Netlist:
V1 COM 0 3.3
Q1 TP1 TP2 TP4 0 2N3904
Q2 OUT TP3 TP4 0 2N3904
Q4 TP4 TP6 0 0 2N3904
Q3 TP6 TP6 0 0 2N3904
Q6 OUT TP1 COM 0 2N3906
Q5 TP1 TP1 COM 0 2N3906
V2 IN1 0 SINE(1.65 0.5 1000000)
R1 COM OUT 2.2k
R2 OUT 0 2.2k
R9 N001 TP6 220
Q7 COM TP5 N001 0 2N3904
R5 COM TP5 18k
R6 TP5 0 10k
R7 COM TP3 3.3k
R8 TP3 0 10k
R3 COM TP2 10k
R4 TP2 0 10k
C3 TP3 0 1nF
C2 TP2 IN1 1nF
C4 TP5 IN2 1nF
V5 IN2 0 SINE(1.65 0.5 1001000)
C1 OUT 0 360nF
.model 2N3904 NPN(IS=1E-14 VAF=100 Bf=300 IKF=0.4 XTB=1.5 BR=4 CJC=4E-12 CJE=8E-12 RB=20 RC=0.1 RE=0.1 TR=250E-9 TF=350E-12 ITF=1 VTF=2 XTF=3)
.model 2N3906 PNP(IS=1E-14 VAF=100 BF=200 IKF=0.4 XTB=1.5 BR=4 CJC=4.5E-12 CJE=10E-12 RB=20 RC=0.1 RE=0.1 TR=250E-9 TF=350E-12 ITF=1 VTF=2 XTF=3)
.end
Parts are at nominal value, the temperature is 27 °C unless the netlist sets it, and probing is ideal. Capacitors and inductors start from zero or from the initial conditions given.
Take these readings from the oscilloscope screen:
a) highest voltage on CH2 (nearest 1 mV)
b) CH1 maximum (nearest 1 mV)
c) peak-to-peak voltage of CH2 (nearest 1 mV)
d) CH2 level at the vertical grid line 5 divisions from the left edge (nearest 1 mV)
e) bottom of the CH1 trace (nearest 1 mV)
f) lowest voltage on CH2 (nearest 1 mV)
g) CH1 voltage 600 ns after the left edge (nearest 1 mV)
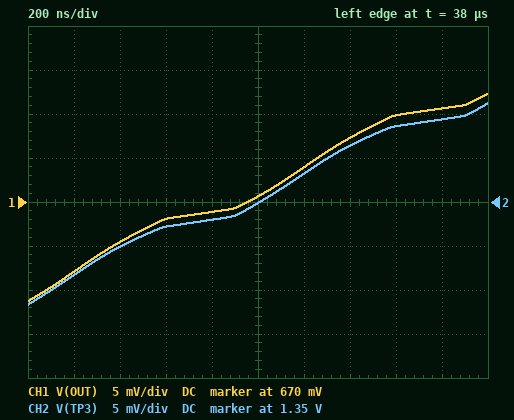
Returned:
1.361 V
682 mV
23 mV
1.350 V
659 mV
1.338 V
668 mV
